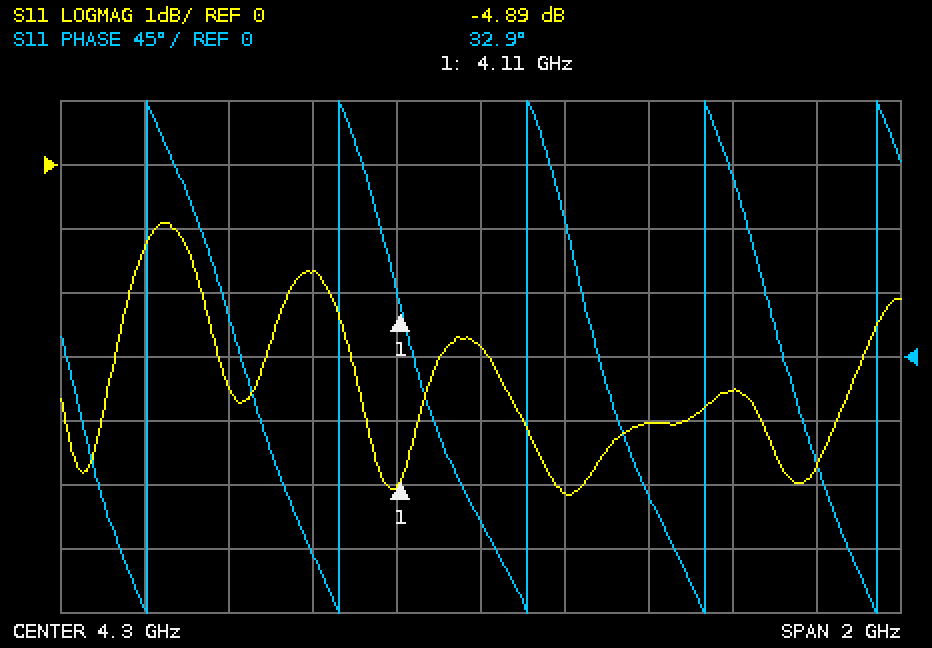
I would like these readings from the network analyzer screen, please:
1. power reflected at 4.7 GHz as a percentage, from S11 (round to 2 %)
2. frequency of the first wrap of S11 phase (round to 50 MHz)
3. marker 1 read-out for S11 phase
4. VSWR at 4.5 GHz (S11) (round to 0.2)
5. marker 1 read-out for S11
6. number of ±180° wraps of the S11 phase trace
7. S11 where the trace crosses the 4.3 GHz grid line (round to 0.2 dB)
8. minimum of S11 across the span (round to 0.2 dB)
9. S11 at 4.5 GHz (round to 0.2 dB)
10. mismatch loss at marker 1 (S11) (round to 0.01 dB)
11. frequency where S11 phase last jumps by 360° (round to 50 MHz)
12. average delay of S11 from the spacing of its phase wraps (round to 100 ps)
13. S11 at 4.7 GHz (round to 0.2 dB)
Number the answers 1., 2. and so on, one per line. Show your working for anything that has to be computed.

1. 10^(-4/10) ≈ 40 %
2. 3.50 GHz
3. 32.9°
4. |Γ| = 10^(-5.2/20) = 0.5495; VSWR = (1 + 0.5495)/(1 − 0.5495) ≈ 3.4
5. -4.89 dB
6. 5
7. -2.8 dB
8. -5.2 dB
9. -5.2 dB
10. −10 log10(1 − 10^(-4.89/10)) ≈ 1.70 dB
11. 5.25 GHz
12. 4 cycles / (5.25 GHz − 3.50 GHz) ≈ 2.3 ns
13. -4.0 dB
